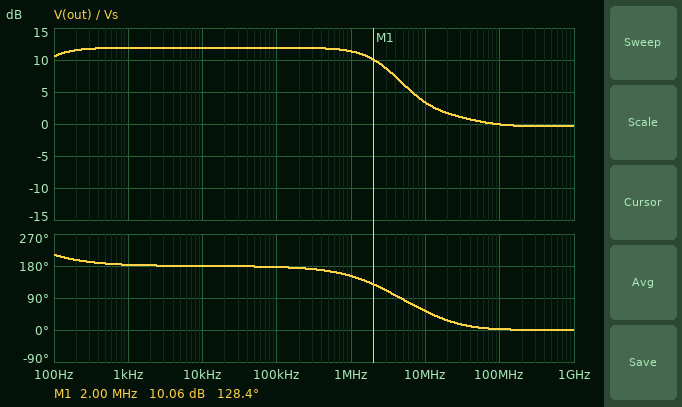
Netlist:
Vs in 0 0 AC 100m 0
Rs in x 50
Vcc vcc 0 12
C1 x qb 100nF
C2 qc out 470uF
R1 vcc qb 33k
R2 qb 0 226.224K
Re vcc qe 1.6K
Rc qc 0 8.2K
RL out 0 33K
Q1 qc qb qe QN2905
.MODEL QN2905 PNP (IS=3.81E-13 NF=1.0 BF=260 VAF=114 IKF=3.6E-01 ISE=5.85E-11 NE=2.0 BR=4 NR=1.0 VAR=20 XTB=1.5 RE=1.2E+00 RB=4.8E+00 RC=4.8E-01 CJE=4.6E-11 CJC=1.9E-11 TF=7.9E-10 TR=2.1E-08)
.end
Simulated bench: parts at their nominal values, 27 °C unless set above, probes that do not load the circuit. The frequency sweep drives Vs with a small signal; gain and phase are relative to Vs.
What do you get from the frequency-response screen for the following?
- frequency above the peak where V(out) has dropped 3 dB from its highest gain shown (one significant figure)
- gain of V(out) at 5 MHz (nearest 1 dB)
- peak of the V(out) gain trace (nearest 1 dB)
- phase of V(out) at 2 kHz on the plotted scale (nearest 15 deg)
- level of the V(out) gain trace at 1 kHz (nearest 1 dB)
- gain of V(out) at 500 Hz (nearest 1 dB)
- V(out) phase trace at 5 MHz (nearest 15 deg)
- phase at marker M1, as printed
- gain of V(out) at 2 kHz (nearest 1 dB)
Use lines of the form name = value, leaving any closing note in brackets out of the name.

frequency above the peak where V(out) has dropped 3 dB from its highest gain shown = 3 MHz
gain of V(out) at 5 MHz = 6 dB
peak of the V(out) gain trace = 12 dB
phase of V(out) at 2 kHz on the plotted scale = 180 deg
level of the V(out) gain trace at 1 kHz = 12 dB
gain of V(out) at 500 Hz = 12 dB
V(out) phase trace at 5 MHz = 90 deg
phase at marker M1, as printed = 128.4 deg
gain of V(out) at 2 kHz = 12 dB
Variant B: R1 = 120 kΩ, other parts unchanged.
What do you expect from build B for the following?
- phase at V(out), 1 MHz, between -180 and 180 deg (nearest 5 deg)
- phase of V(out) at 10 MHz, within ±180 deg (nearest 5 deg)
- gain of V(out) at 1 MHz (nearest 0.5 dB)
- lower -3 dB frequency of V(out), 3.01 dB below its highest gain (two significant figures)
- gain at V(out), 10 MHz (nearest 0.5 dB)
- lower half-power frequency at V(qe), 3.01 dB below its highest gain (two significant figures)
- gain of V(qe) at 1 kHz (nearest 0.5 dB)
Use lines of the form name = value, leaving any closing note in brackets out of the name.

phase at V(out), 1 MHz, between -180 and 180 deg = 70 deg
phase of V(out) at 10 MHz, within ±180 deg = 10 deg
gain of V(out) at 1 MHz = -5.0 dB
lower -3 dB frequency of V(out), 3.01 dB below its highest gain = 1.4 MHz
gain at V(out), 10 MHz = -0.5 dB
lower half-power frequency at V(qe), 3.01 dB below its highest gain = 980 Hz
gain of V(qe) at 1 kHz = -3.5 dB
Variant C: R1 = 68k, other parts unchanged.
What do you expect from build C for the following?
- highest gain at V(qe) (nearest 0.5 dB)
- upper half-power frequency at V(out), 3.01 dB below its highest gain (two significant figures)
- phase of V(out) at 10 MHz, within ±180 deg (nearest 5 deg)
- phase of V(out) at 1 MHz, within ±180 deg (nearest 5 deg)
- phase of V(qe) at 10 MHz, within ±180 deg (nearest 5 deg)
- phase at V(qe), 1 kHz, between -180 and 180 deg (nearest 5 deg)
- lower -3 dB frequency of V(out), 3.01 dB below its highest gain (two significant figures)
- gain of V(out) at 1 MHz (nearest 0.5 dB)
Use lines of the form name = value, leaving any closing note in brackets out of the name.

highest gain at V(qe) = 0 dB
upper half-power frequency at V(out), 3.01 dB below its highest gain = 1.5 MHz
phase of V(out) at 10 MHz, within ±180 deg = 35 deg
phase of V(out) at 1 MHz, within ±180 deg = 135 deg
phase of V(qe) at 10 MHz, within ±180 deg = 0 deg
phase at V(qe), 1 kHz, between -180 and 180 deg = 0 deg
lower -3 dB frequency of V(out), 3.01 dB below its highest gain = 36 Hz
gain of V(out) at 1 MHz = 10.5 dB
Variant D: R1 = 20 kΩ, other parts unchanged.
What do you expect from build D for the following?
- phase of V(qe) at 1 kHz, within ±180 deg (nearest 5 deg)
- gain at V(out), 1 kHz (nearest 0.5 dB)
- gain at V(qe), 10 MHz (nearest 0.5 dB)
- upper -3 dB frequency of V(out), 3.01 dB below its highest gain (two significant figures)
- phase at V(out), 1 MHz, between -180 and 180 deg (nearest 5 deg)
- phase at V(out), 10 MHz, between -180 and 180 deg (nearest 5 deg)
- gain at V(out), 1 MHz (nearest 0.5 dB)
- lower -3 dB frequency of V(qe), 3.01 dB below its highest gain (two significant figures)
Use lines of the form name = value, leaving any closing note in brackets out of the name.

phase of V(qe) at 1 kHz, within ±180 deg = 5 deg
gain at V(out), 1 kHz = 11.5 dB
gain at V(qe), 10 MHz = -1.0 dB
upper -3 dB frequency of V(out), 3.01 dB below its highest gain = 3.2 MHz
phase at V(out), 1 MHz, between -180 and 180 deg = 155 deg
phase at V(out), 10 MHz, between -180 and 180 deg = 50 deg
gain at V(out), 1 MHz = 11.0 dB
lower -3 dB frequency of V(qe), 3.01 dB below its highest gain = 97 Hz
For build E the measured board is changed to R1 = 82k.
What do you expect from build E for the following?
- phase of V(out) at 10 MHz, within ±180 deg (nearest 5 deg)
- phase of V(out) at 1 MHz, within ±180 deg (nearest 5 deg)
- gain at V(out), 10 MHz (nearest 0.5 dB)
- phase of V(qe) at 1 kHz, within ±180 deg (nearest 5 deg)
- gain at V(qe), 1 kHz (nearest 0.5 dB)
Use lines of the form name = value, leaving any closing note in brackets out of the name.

phase of V(out) at 10 MHz, within ±180 deg = 20 deg
phase of V(out) at 1 MHz, within ±180 deg = 115 deg
gain at V(out), 10 MHz = 0 dB
phase of V(qe) at 1 kHz, within ±180 deg = 30 deg
gain at V(qe), 1 kHz = -1.5 dB
